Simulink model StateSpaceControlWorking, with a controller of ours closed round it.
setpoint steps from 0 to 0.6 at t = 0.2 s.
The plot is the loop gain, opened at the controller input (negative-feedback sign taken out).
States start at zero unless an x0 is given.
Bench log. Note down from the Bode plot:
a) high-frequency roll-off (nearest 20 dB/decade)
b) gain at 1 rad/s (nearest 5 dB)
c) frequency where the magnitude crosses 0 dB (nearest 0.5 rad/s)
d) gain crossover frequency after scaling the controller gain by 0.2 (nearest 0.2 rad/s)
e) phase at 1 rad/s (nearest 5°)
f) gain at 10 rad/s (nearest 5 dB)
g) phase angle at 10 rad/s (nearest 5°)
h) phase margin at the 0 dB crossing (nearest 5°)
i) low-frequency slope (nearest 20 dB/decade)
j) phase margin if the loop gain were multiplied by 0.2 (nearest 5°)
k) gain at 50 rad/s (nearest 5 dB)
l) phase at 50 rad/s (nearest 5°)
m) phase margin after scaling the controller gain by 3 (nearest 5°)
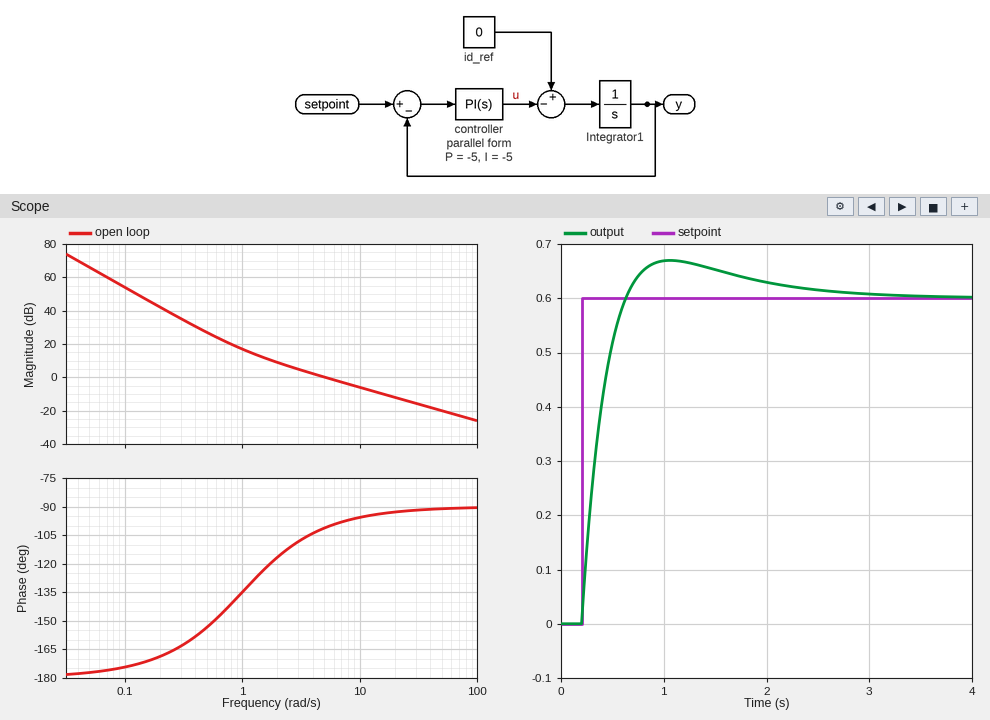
-20 dB/decade
15 dB
5.0 rad/s
1.2 rad/s
-135°
-5 dB
-95°
80°
-40 dB/decade
50°
-20 dB
-90°
85°
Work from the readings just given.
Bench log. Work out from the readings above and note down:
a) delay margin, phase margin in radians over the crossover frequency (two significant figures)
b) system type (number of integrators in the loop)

0.28 s
2
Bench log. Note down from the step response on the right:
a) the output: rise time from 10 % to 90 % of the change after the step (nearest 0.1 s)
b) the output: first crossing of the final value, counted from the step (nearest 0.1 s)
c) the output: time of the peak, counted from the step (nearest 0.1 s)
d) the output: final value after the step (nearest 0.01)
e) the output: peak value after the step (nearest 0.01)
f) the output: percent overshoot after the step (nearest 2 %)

0.3 s
0.4 s
0.9 s
0.60
0.67
12 %
